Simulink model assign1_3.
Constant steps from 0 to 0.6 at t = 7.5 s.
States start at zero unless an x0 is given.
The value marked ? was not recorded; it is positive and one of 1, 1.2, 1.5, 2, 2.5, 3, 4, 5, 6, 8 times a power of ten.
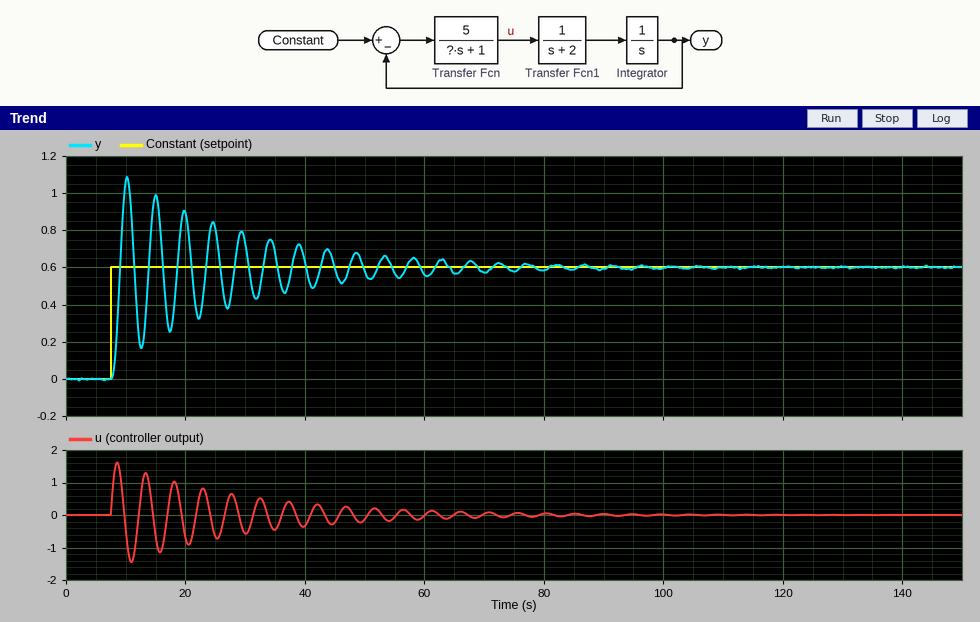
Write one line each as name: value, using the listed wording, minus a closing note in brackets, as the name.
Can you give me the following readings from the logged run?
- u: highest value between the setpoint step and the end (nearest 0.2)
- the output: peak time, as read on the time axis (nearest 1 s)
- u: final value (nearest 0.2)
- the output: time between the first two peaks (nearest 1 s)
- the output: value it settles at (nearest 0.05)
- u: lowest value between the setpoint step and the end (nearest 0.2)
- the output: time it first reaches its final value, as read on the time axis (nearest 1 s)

u: highest value between the setpoint step and the end: 1.6
the output: peak time, as read on the time axis: 10 s
u: final value: 0.0
the output: time between the first two peaks: 5 s
the output: value it settles at: 0.60
u: lowest value between the setpoint step and the end: -1.4
the output: time it first reaches its final value, as read on the time axis: 9 s
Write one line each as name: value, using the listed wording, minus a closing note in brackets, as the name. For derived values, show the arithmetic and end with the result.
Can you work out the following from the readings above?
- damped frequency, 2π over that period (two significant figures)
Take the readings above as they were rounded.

damped frequency, 2π over that period: 2π / 5 = 1.3 rad/s
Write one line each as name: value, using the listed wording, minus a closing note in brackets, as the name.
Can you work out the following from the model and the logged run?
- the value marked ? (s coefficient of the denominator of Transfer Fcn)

the value marked ?: 1
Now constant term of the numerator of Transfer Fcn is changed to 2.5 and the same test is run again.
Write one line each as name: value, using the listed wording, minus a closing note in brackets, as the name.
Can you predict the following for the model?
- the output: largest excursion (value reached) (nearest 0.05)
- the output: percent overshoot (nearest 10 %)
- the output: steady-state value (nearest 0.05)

the output: largest excursion (value reached): 0.90
the output: percent overshoot: 50 %
the output: steady-state value: 0.60
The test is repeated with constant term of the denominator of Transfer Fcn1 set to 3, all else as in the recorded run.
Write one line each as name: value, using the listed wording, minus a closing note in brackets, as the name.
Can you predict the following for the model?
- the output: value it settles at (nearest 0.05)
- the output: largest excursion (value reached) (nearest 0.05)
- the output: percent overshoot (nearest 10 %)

the output: value it settles at: 0.60
the output: largest excursion (value reached): 0.90
the output: percent overshoot: 50 %
